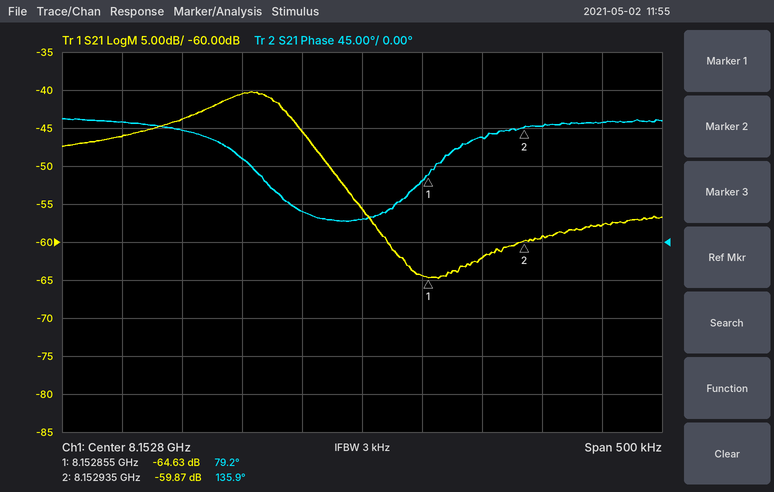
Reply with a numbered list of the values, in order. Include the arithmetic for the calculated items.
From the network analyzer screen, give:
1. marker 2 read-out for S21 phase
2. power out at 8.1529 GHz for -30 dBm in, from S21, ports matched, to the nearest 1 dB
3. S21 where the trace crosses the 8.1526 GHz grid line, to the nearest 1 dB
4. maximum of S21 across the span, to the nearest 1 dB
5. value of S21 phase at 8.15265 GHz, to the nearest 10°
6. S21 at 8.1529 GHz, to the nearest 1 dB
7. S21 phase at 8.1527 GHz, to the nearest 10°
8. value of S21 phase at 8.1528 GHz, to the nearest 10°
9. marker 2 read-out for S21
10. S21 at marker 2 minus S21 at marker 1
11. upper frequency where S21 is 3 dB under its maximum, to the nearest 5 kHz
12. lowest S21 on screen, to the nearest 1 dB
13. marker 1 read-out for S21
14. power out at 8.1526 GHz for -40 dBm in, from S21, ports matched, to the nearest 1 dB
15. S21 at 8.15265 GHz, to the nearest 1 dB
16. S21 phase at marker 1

1. 135.9°
2. -30 dBm + (-62 dB) = -92 dBm
3. -46 dB
4. -40 dB
5. 130°
6. -62 dB
7. 100°
8. 30°
9. -59.87 dB
10. -59.87 − (-64.63) = 4.76 dB
11. 8.152740 GHz
12. -65 dB
13. -64.63 dB
14. -40 dBm + (-46 dB) = -86 dBm
15. -44 dB
16. 79.2°
